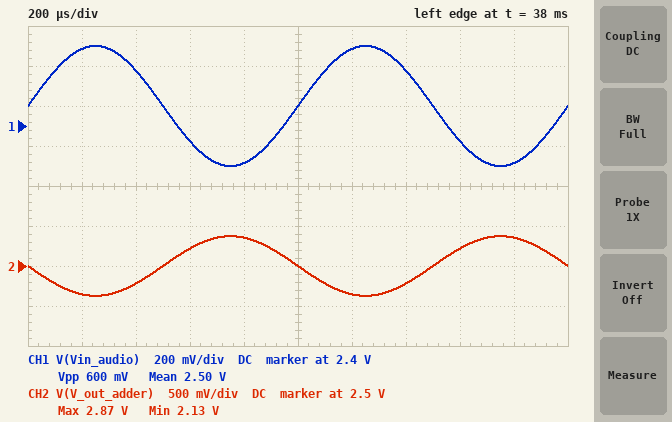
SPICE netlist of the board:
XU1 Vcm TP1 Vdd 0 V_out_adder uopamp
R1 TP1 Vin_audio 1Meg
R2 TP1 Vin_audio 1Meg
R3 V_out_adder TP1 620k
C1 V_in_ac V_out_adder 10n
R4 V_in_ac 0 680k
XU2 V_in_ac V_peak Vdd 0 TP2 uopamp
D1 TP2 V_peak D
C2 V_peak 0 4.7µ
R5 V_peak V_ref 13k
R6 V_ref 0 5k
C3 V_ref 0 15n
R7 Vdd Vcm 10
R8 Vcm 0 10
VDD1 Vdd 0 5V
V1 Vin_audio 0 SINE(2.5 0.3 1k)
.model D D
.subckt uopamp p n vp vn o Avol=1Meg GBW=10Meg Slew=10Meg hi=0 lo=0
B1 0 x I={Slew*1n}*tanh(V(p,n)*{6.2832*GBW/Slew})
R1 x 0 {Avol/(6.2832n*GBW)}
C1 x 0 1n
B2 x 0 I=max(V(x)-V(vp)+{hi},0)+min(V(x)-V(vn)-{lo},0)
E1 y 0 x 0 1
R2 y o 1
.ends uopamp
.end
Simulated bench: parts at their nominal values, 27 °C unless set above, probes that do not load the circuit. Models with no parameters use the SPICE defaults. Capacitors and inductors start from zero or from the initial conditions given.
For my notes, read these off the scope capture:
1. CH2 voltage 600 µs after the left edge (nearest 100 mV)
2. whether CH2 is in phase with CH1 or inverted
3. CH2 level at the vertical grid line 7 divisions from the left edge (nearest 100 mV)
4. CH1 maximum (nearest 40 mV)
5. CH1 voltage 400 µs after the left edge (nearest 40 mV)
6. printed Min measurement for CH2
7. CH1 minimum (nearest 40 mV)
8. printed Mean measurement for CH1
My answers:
2.7 V
inverted
2.3 V
2.80 V
2.68 V
2.13 V
2.20 V
2.50 V
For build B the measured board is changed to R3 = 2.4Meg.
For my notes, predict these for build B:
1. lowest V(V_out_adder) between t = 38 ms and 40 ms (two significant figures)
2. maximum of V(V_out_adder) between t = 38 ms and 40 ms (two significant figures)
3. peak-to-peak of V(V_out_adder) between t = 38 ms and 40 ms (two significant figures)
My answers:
1.1 V
3.9 V
2.9 V
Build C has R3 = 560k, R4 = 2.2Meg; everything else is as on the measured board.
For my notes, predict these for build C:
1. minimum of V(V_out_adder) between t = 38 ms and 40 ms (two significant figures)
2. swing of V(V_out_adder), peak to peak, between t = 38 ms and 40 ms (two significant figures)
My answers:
2.2 V
670 mV
